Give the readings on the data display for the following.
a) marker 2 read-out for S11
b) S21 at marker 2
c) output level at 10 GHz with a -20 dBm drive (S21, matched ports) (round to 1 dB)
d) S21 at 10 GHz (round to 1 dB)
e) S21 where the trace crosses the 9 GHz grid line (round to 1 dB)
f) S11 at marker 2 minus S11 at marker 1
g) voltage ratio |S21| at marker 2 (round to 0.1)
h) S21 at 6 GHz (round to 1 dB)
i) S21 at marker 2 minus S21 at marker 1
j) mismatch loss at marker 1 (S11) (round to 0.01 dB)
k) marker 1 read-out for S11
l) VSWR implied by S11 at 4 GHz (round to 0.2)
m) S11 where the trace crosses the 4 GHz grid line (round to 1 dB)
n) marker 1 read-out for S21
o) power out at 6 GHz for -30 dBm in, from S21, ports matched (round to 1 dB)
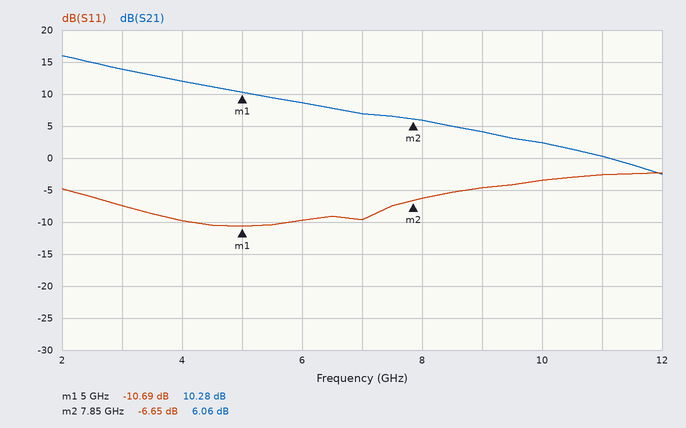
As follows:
-6.65 dB
6.06 dB
-18 dBm
2 dB
4 dB
4.04 dB
2.0
9 dB
-4.22 dB
0.39 dB
-10.69 dB
2.0
-10 dB
10.28 dB
-21 dBm
